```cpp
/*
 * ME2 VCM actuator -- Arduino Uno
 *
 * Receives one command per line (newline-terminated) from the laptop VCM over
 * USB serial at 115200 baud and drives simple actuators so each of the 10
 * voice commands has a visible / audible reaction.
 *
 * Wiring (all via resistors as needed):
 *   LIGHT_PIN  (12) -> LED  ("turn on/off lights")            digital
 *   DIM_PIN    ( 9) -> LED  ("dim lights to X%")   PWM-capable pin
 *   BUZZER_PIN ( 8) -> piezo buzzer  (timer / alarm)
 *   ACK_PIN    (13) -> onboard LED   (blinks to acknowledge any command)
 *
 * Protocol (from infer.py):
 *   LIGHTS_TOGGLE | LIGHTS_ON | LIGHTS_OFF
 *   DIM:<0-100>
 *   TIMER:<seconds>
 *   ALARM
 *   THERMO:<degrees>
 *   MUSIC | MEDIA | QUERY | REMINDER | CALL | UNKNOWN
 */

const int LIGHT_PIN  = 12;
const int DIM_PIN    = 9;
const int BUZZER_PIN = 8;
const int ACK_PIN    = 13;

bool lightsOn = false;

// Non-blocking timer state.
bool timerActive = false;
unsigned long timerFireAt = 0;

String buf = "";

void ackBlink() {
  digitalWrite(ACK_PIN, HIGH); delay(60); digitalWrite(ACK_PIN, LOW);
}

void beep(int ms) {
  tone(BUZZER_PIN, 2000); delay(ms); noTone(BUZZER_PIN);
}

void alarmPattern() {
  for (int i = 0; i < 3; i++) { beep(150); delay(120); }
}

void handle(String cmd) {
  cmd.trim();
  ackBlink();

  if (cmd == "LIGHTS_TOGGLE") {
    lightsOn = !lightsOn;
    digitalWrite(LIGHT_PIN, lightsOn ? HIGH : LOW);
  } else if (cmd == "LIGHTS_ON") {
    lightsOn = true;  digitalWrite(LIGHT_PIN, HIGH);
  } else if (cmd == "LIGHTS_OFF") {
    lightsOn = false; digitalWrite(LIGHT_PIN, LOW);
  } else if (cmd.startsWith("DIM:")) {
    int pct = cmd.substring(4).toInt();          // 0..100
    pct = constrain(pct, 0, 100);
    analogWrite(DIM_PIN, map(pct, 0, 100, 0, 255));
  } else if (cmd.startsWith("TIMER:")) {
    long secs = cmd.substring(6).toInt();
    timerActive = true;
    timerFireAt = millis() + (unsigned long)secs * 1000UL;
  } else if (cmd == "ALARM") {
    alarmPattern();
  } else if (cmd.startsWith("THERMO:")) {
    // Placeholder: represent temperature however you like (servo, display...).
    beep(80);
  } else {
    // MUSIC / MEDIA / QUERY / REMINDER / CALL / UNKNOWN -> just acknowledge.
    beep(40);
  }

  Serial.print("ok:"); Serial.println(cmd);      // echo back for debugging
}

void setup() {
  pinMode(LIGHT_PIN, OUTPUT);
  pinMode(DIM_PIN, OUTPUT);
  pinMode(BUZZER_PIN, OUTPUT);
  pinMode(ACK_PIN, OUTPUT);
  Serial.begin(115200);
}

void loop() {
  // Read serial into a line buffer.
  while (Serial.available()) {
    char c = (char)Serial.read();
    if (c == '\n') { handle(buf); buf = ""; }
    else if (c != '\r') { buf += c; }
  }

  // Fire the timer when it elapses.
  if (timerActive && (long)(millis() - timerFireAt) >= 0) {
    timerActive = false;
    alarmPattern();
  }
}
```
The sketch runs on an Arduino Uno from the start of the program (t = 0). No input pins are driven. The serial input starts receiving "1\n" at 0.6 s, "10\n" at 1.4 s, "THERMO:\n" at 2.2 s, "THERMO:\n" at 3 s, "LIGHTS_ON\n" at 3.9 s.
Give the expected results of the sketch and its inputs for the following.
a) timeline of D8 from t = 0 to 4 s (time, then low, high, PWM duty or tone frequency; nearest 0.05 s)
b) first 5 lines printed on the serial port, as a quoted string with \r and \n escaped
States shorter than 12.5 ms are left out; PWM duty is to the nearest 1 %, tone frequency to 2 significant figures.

0 s low; 0.65 s tone 2000 Hz; 0.7 s low; 1.45 s tone 2000 Hz; 1.5 s low; 2.25 s tone 2000 Hz; 2.35 s low; 3.05 s tone 2000 Hz; 3.15 s low
"ok:1\r\nok:10\r\nok:THERMO:\r\nok:THERMO:\r\nok:LIGHTS_ON\r\n"
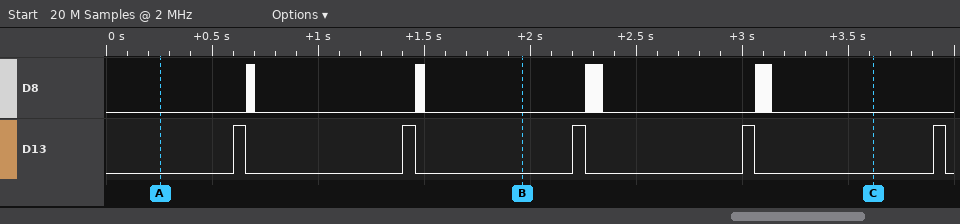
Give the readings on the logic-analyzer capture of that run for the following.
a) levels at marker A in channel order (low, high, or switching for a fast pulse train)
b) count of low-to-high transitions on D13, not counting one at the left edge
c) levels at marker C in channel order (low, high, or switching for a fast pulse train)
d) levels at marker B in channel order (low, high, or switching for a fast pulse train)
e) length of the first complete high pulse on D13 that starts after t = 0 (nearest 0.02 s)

D8 low, D13 low
5
D8 low, D13 low
D8 low, D13 low
0.06 s
